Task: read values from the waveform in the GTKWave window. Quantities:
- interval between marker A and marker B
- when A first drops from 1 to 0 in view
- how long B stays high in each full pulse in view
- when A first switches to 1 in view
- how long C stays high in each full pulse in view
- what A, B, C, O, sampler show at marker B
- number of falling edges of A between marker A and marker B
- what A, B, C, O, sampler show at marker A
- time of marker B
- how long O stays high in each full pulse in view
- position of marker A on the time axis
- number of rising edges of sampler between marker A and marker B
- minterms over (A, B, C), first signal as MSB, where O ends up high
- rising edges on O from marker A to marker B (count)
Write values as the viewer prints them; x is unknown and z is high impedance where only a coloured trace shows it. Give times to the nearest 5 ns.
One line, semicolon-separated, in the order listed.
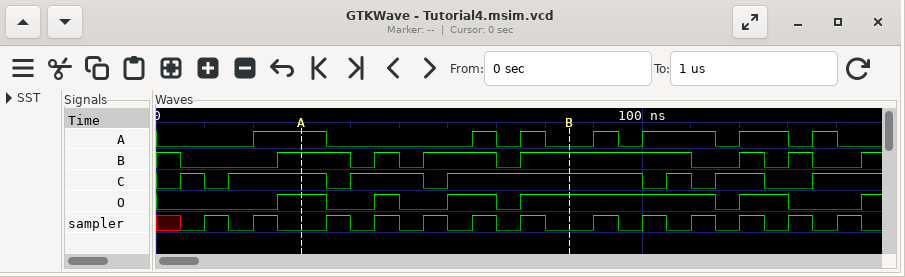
55 ns; 35 ns; 15 ns, 5 ns, 15 ns, 35 ns, 5 ns, 5 ns; 20 ns; 5 ns, 20 ns, 15 ns, 40 ns, 5 ns, 10 ns; A=0, B=1, C=1, O=1, sampler=0; 3; A=1, B=1, C=1, O=1, sampler=0; 85 ns; 10 ns, 5 ns, 10 ns, 40 ns, 10 ns; 30 ns; 5; 3, 4, 6, 7; 3
